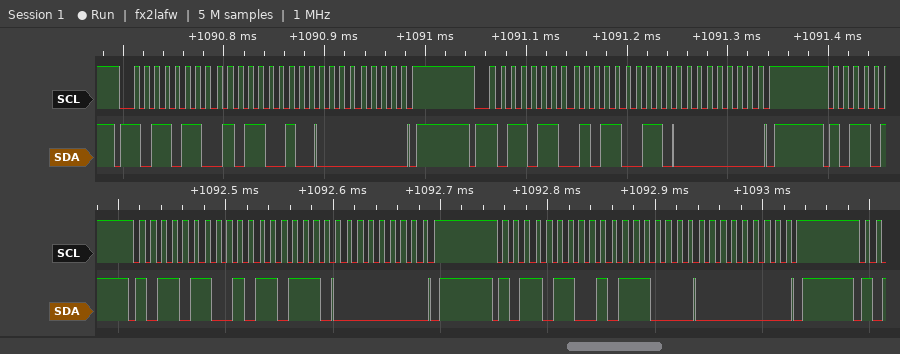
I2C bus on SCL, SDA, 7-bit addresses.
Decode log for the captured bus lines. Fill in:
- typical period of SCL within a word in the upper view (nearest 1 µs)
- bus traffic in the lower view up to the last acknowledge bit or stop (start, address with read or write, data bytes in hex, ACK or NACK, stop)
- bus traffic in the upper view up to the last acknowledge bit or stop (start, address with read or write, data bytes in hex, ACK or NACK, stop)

10 µs
start, address 5B write ACK, B7 ACK, 00 ACK, stop, start, address 5B write ACK, B8 ACK, 00 ACK, stop
start, address 5B write ACK, B2 ACK, 00 ACK, stop, start, address 5B write ACK, B3 ACK, 00 ACK, stop
